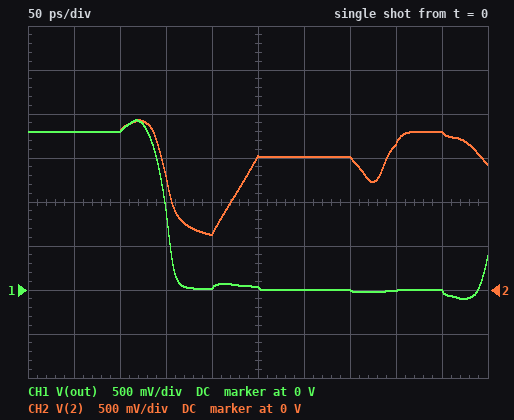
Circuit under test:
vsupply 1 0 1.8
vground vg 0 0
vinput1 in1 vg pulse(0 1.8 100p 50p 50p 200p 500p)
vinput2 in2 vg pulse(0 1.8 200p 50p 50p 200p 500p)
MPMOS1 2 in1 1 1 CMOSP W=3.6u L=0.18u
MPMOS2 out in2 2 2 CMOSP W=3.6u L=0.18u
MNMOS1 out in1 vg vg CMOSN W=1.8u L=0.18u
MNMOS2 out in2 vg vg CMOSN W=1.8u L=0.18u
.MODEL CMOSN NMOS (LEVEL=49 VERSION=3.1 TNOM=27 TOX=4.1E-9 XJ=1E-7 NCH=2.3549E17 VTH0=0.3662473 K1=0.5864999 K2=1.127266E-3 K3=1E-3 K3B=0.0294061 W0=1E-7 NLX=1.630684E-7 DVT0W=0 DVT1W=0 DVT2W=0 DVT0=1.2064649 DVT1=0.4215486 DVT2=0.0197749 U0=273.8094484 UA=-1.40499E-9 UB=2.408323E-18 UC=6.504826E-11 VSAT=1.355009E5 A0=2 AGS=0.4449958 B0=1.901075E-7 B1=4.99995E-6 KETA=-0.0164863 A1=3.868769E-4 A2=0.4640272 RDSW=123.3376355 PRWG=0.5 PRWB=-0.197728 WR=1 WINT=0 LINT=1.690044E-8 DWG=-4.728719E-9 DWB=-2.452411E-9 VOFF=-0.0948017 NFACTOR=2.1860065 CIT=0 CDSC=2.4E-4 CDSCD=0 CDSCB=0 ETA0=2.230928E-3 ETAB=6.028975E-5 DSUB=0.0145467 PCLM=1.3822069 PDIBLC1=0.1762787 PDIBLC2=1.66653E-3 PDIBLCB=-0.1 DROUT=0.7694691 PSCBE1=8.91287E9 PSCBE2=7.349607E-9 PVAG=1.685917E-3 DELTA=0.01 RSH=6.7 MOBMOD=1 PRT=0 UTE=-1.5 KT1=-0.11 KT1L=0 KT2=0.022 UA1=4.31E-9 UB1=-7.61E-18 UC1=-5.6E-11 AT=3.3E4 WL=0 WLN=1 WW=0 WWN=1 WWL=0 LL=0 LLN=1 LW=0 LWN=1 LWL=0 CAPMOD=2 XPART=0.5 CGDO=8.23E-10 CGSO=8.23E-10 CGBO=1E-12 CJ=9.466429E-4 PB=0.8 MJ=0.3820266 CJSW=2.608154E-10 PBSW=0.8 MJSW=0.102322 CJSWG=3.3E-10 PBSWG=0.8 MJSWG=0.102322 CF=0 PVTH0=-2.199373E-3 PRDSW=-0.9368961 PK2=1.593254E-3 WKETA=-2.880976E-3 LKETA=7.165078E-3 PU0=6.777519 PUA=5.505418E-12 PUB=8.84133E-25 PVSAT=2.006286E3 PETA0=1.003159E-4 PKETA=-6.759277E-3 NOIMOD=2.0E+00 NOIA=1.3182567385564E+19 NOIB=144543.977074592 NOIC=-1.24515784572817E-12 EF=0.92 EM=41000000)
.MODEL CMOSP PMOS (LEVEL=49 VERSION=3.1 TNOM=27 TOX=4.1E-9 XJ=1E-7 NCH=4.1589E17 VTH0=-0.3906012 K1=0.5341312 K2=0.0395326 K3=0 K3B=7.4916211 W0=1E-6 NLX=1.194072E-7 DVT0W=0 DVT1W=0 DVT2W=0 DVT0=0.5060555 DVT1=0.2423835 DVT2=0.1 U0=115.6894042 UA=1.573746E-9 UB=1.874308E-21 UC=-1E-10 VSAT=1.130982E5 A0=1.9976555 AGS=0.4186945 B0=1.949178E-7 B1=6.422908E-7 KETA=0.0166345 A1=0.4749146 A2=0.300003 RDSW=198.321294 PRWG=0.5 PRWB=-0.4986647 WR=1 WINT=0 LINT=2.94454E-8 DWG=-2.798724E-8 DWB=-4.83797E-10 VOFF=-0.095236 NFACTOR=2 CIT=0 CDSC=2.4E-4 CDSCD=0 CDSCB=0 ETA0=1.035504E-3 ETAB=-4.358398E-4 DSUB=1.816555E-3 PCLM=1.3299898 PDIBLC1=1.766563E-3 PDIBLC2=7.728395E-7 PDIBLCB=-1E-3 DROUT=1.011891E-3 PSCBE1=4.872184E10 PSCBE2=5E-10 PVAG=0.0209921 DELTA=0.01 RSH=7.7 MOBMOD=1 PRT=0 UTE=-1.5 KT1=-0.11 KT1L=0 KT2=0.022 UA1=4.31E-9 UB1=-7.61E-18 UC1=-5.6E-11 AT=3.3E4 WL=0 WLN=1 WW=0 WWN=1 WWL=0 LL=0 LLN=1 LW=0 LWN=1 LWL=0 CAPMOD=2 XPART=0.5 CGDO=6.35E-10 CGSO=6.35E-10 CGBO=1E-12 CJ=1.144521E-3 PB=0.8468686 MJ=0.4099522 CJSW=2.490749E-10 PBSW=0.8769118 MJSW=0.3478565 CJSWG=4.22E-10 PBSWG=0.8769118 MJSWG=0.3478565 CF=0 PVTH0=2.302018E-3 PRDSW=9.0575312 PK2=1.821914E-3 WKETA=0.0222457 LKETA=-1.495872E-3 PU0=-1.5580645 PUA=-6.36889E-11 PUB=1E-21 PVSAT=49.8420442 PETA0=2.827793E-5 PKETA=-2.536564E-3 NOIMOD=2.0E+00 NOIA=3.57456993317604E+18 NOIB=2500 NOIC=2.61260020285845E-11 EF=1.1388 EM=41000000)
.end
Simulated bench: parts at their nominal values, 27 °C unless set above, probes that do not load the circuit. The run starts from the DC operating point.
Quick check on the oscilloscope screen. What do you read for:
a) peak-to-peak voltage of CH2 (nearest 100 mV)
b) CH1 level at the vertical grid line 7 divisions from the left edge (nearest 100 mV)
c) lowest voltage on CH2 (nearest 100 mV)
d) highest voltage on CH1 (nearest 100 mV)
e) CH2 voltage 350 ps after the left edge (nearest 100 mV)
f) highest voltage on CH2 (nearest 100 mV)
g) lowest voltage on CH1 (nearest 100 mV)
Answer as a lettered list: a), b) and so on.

a) 1.3 V
b) 0 V
c) 600 mV
d) 1.9 V
e) 1.5 V
f) 1.9 V
g) -100 mV
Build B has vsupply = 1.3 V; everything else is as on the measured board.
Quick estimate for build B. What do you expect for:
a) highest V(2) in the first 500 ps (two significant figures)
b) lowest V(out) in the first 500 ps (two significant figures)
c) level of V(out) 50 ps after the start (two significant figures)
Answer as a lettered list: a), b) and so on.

a) 1.5 V
b) -290 mV
c) 1.3 V
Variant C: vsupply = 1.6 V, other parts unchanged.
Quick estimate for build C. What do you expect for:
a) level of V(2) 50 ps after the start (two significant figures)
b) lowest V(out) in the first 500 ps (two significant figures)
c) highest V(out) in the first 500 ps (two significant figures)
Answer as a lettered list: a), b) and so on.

a) 1.6 V
b) -140 mV
c) 1.7 V
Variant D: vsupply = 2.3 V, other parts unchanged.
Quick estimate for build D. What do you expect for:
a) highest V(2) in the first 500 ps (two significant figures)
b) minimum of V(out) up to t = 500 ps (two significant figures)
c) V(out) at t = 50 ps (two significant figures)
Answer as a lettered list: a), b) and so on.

a) 2.4 V
b) -71 mV
c) 2.3 V
